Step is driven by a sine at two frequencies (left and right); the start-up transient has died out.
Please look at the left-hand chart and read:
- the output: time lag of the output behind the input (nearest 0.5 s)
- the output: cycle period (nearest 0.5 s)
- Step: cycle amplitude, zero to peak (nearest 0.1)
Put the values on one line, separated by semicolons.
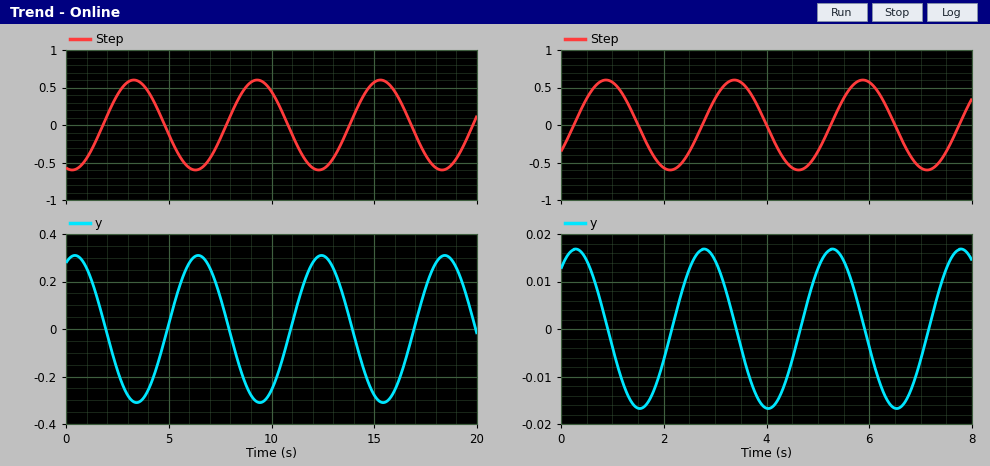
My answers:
3.0 s; 6.0 s; 0.6
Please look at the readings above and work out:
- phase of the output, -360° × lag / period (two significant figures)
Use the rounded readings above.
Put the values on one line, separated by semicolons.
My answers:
-180°
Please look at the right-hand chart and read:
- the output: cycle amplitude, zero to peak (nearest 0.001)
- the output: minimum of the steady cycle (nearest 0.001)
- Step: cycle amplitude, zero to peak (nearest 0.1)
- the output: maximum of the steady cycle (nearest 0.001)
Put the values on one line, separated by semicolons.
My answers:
0.017; -0.017; 0.6; 0.017
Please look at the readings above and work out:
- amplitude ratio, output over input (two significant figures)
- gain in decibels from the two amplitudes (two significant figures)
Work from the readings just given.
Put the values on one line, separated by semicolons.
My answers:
0.028; -31 dB
